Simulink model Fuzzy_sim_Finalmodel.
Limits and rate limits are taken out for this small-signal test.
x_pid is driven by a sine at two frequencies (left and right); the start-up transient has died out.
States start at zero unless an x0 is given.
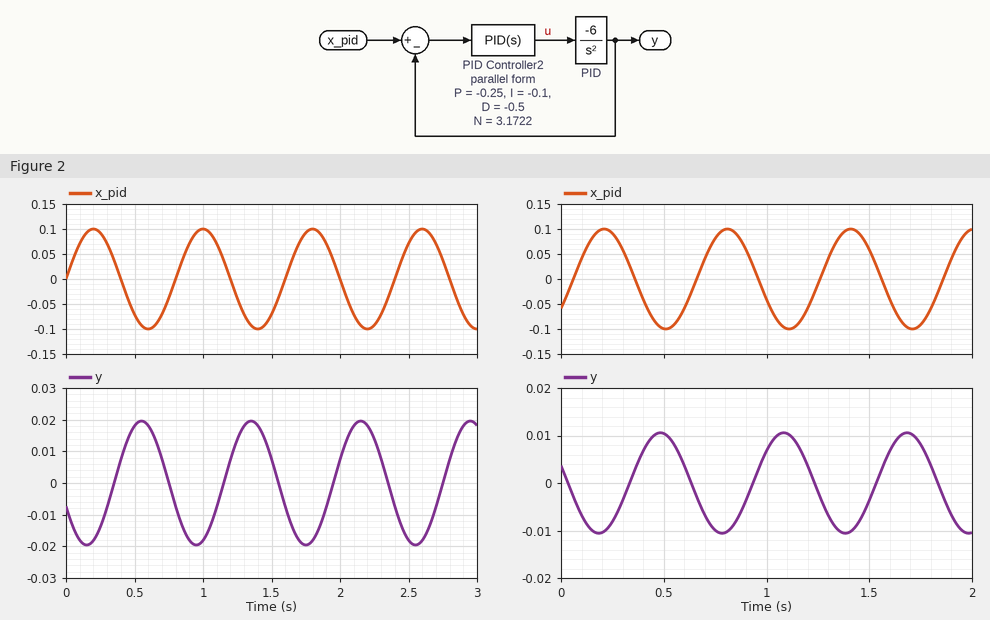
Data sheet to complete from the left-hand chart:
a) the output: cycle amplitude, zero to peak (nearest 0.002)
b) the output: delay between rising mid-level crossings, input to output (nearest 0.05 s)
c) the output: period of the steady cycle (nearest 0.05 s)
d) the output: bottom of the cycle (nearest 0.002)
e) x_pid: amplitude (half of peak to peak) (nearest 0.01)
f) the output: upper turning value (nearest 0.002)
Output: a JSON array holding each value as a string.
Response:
["0.020", "0.35 s", "0.80 s", "-0.020", "0.10", "0.020"]
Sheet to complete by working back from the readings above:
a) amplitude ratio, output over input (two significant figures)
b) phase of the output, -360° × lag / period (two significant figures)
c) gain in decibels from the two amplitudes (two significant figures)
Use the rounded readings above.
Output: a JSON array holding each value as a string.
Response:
["0.20", "-160°", "-14 dB"]
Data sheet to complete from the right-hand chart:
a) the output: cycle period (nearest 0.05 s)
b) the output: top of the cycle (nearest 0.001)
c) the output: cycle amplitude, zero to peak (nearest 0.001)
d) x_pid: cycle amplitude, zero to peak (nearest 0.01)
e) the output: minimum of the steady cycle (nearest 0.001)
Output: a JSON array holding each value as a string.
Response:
["0.60 s", "0.011", "0.011", "0.10", "-0.011"]
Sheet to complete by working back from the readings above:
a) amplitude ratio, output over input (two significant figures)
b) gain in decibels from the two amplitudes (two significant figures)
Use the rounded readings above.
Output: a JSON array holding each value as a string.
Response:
["0.11", "-19 dB"]
